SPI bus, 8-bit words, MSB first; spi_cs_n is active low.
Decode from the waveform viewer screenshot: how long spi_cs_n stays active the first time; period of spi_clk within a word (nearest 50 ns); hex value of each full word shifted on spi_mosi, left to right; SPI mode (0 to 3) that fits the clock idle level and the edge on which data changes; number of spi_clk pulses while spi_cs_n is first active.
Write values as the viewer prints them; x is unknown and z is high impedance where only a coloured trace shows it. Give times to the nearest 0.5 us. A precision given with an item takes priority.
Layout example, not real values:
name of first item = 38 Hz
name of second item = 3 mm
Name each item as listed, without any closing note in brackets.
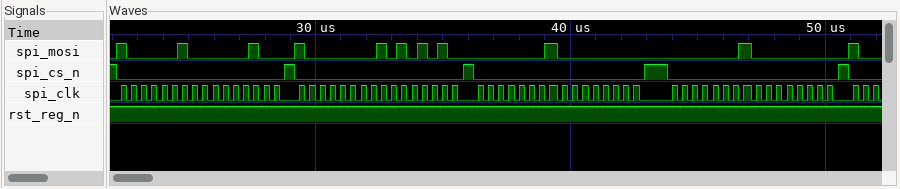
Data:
how long spi_cs_n stays active the first time = 6.5 us
period of spi_clk within a word = 400 ns
hex value of each full word shifted on spi_mosi, left to right = 82, 04, 80, AA, 01, 00, 01, 00
SPI mode (0 to 3) that fits the clock idle level and the edge on which data changes = 0
number of spi_clk pulses while spi_cs_n is first active = 16
